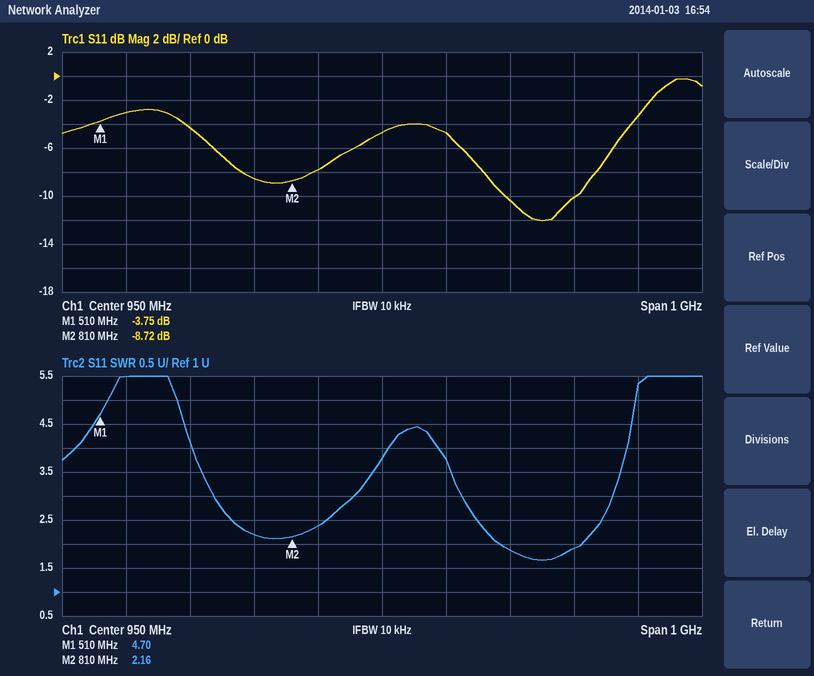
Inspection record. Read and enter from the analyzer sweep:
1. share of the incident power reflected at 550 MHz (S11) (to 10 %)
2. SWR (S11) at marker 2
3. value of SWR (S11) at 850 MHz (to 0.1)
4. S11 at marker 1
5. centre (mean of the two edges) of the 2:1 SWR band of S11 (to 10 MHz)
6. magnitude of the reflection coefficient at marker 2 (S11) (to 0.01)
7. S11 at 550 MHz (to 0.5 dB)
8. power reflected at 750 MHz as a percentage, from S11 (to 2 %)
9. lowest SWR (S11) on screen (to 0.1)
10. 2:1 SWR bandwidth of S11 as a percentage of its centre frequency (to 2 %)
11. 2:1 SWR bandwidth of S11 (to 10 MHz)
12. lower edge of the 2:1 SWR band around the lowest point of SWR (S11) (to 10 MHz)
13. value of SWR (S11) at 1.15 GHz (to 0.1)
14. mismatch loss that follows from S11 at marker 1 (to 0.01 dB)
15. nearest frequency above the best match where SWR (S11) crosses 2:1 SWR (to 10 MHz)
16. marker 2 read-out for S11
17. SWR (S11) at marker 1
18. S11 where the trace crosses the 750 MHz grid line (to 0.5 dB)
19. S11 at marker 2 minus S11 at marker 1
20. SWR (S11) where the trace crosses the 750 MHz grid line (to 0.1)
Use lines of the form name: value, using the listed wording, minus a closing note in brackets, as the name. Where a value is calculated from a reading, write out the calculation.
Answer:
share of the incident power reflected at 550 MHz (S11): 10^(-3/10) ≈ 50 %
SWR (S11) at marker 2: 2.16
value of SWR (S11) at 850 MHz: 2.4
S11 at marker 1: -3.75 dB
centre (mean of the two edges) of the 2:1 SWR band of S11: 1.20 GHz
magnitude of the reflection coefficient at marker 2 (S11): 10^(-8.72/20) ≈ 0.37
S11 at 550 MHz: -3.0 dB
power reflected at 750 MHz as a percentage, from S11: 10^(-8.5/10) ≈ 14 %
lowest SWR (S11) on screen: 1.7
2:1 SWR bandwidth of S11 as a percentage of its centre frequency: 130 MHz / 1.195 GHz ≈ 10.9 %, so 10 % to the nearest 2 %
2:1 SWR bandwidth of S11: 1.26 GHz − 1.13 GHz = 130 MHz
lower edge of the 2:1 SWR band around the lowest point of SWR (S11): 1.13 GHz
value of SWR (S11) at 1.15 GHz: 1.9
mismatch loss that follows from S11 at marker 1: −10 log10(1 − 10^(-3.75/10)) ≈ 2.38 dB
nearest frequency above the best match where SWR (S11) crosses 2:1 SWR: 1.26 GHz
marker 2 read-out for S11: -8.72 dB
SWR (S11) at marker 1: 4.70
S11 where the trace crosses the 750 MHz grid line: -8.5 dB
S11 at marker 2 minus S11 at marker 1: -8.72 − (-3.75) = -4.97 dB
SWR (S11) where the trace crosses the 750 MHz grid line: 2.2
